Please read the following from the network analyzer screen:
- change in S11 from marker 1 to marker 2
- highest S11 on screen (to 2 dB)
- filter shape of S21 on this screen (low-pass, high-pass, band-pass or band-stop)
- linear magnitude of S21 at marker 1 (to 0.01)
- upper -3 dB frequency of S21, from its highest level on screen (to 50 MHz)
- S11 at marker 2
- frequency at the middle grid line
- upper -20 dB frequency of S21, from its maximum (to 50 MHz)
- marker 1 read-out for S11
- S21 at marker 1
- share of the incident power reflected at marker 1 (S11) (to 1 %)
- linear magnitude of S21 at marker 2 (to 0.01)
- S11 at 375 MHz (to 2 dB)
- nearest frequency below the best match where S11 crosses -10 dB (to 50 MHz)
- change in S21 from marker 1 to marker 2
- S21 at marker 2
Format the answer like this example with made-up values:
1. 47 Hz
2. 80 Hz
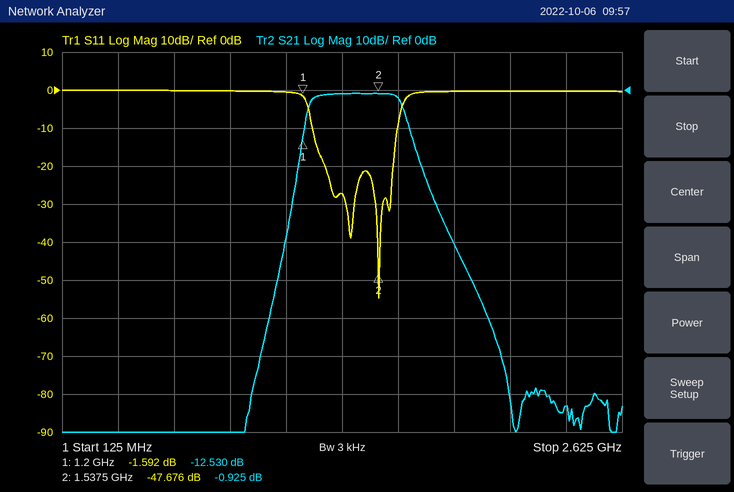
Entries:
1. -46.084 dB
2. 0 dB
3. band-pass
4. 0.24
5. 1.65 GHz
6. -47.676 dB
7. 1.375 GHz
8. 1.75 GHz
9. -1.592 dB
10. -12.530 dB
11. 69 %
12. 0.90
13. 0 dB
14. 1.25 GHz
15. 11.605 dB
16. -0.925 dB
